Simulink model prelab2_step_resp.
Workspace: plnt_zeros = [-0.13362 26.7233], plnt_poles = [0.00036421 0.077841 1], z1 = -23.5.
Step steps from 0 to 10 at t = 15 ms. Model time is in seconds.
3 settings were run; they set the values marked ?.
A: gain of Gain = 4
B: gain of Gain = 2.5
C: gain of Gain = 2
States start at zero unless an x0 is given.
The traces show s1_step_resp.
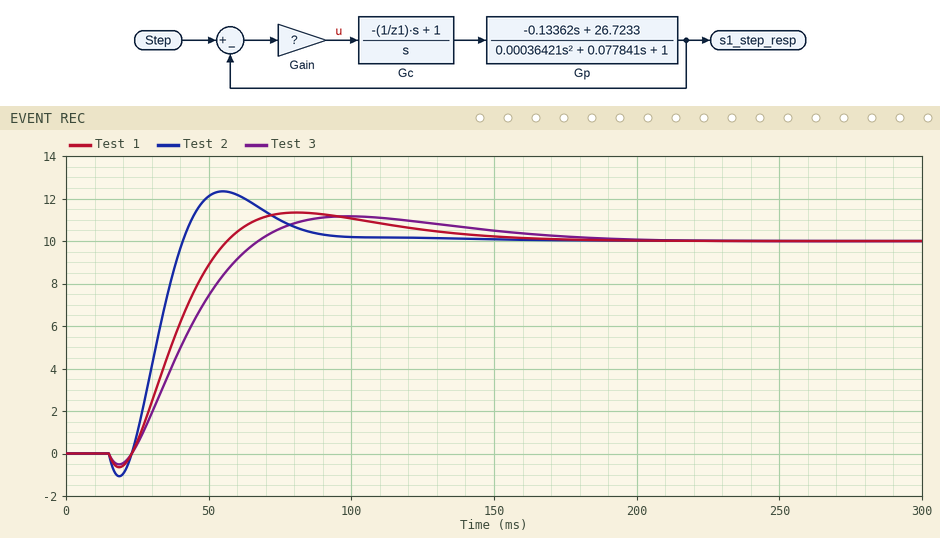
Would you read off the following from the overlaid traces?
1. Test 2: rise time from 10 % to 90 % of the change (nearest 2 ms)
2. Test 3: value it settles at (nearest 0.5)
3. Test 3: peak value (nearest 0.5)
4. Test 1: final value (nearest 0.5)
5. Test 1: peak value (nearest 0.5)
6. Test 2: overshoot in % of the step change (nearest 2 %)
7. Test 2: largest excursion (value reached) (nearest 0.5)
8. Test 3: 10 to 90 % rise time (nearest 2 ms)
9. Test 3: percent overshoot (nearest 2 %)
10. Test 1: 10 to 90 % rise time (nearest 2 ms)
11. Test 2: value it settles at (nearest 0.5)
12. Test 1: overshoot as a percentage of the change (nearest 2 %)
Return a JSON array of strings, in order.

["14 ms", "10.0", "11.0", "10.0", "11.5", "24 %", "12.5", "32 ms", "12 %", "24 ms", "10.0", "14 %"]
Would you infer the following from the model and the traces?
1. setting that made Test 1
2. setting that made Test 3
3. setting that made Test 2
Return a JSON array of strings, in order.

["B", "C", "A"]
